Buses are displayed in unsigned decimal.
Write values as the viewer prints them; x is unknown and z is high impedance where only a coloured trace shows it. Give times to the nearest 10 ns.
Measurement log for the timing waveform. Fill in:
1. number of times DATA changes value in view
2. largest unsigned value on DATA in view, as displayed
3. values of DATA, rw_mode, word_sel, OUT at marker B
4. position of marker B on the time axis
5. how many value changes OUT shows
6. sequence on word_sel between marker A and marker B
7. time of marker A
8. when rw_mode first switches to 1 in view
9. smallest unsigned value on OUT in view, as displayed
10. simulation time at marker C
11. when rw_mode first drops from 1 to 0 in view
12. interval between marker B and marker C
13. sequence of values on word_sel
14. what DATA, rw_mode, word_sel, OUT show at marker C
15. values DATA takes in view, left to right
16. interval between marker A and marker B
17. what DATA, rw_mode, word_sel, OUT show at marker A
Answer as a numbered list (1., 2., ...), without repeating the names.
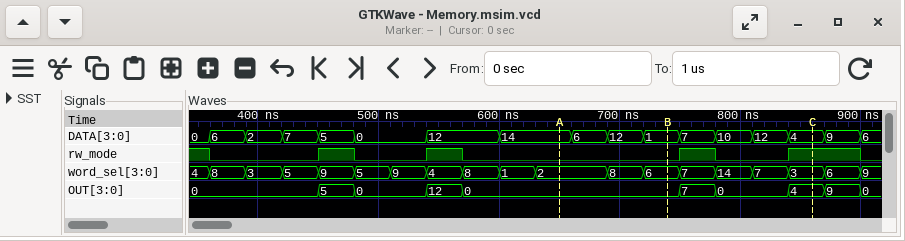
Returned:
1. 16
2. 14
3. DATA=1, rw_mode=0, word_sel=6, OUT=0
4. 740 ns
5. 9
6. 2, 8, 6
7. 650 ns
8. 450 ns
9. 0
10. 860 ns
11. 360 ns
12. 120 ns
13. 4, 8, 3, 5, 9, 5, 9, 4, 8, 1, 2, 8, 6, 7, 14, 7, 3, 6, 9
14. DATA=4, rw_mode=1, word_sel=3, OUT=4
15. 0, 6, 2, 7, 5, 0, 12, 14, 6, 12, 1, 7, 10, 12, 4, 9, 6
16. 90 ns
17. DATA=14, rw_mode=0, word_sel=2, OUT=0
